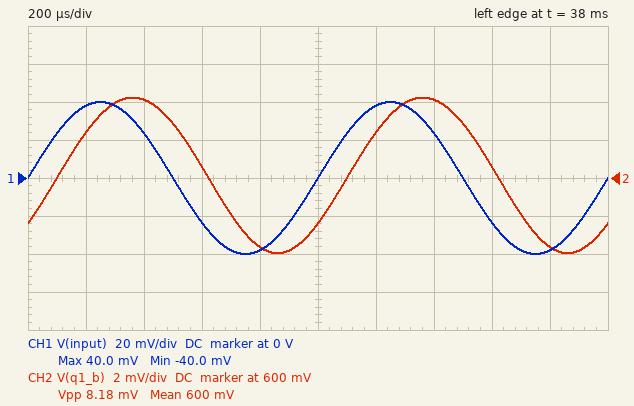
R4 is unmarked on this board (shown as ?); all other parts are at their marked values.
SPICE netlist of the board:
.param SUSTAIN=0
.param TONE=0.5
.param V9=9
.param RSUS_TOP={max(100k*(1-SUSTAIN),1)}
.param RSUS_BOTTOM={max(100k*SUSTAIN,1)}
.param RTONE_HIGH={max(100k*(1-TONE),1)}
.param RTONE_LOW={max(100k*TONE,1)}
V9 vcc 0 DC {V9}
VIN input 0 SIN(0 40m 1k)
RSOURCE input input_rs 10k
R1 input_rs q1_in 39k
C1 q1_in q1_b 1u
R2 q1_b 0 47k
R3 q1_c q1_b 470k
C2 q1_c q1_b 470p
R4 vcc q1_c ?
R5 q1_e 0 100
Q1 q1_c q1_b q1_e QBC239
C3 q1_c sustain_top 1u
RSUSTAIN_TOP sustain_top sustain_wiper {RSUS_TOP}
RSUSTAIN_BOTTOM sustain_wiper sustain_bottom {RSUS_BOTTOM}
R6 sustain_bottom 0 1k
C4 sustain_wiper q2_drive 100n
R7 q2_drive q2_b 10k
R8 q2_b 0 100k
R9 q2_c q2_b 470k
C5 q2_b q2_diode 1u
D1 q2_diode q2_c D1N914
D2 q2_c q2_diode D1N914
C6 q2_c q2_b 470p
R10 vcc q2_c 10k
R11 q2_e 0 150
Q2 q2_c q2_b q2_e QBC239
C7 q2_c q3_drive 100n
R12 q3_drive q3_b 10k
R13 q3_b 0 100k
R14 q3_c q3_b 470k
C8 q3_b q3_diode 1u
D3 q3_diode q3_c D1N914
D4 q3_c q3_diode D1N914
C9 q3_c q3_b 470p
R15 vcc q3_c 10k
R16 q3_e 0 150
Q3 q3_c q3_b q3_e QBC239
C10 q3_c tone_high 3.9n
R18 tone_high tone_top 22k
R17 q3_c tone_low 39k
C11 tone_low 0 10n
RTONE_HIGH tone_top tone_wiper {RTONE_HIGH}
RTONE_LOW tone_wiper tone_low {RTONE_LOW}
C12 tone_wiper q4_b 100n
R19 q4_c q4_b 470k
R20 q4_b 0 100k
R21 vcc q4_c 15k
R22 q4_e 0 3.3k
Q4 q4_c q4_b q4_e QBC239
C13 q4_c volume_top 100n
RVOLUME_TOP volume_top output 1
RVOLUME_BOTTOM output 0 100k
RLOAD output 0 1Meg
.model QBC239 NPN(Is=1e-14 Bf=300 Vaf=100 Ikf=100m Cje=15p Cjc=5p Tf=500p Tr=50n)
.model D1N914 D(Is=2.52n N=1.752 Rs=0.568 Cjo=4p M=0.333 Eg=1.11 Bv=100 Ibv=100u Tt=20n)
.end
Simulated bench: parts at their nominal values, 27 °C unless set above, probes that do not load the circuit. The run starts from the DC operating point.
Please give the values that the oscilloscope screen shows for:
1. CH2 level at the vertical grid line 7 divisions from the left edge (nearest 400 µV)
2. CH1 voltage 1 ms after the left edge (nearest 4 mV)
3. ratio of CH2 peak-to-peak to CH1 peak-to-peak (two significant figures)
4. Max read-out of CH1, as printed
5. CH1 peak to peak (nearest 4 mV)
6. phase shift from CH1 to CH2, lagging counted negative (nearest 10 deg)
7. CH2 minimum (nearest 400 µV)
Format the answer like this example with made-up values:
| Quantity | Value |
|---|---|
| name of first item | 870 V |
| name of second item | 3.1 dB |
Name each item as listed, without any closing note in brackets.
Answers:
| Quantity | Value |
|---|---|
| CH2 level at the vertical grid line 7 divisions from the left edge | 604.0 mV |
| CH1 voltage 1 ms after the left edge | 0 V |
| ratio of CH2 peak-to-peak to CH1 peak-to-peak | 0.10 |
| Max read-out of CH1, as printed | 40.0 mV |
| CH1 peak to peak | 80 mV |
| phase shift from CH1 to CH2, lagging counted negative | -40 deg |
| CH2 minimum | 596.0 mV |
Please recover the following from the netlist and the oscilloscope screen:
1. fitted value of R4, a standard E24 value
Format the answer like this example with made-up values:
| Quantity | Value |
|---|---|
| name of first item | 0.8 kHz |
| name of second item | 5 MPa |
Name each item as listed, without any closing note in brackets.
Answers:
| Quantity | Value |
|---|---|
| fitted value of R4, a standard E24 value | 22 kΩ |
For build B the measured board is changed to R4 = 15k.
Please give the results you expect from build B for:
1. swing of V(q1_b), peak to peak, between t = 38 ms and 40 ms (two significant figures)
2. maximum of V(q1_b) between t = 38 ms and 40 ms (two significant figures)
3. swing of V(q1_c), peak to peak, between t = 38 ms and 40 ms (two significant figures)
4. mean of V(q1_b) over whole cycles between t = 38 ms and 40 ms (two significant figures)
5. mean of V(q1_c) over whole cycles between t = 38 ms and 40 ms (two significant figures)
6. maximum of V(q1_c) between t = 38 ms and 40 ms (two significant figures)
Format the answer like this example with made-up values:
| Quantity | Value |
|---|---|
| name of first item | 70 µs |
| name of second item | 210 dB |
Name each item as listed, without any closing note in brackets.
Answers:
| Quantity | Value |
|---|---|
| swing of V(q1_b), peak to peak, between t = 38 ms and 40 ms | 8.6 mV |
| maximum of V(q1_b) between t = 38 ms and 40 ms | 620 mV |
| swing of V(q1_c), peak to peak, between t = 38 ms and 40 ms | 350 mV |
| mean of V(q1_b) over whole cycles between t = 38 ms and 40 ms | 610 mV |
| mean of V(q1_c) over whole cycles between t = 38 ms and 40 ms | 6.9 V |
| maximum of V(q1_c) between t = 38 ms and 40 ms | 7.1 V |
